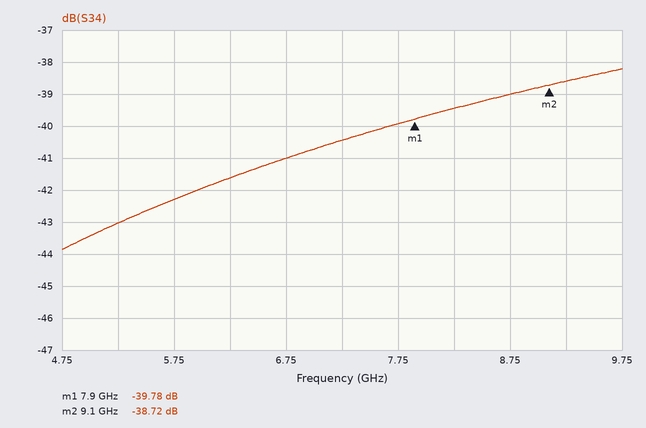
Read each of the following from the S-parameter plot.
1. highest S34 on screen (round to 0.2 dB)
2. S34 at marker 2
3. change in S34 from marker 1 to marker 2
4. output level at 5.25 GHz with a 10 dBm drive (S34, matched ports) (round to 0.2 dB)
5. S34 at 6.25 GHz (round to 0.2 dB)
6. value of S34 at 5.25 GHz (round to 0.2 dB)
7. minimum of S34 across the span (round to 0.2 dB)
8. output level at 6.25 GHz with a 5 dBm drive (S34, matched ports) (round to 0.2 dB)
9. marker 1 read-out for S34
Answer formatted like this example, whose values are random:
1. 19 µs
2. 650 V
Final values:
1. -38.2 dB
2. -38.72 dB
3. 1.06 dB
4. -33.0 dBm
5. -41.6 dB
6. -43.0 dB
7. -43.8 dB
8. -36.6 dBm
9. -39.78 dB
